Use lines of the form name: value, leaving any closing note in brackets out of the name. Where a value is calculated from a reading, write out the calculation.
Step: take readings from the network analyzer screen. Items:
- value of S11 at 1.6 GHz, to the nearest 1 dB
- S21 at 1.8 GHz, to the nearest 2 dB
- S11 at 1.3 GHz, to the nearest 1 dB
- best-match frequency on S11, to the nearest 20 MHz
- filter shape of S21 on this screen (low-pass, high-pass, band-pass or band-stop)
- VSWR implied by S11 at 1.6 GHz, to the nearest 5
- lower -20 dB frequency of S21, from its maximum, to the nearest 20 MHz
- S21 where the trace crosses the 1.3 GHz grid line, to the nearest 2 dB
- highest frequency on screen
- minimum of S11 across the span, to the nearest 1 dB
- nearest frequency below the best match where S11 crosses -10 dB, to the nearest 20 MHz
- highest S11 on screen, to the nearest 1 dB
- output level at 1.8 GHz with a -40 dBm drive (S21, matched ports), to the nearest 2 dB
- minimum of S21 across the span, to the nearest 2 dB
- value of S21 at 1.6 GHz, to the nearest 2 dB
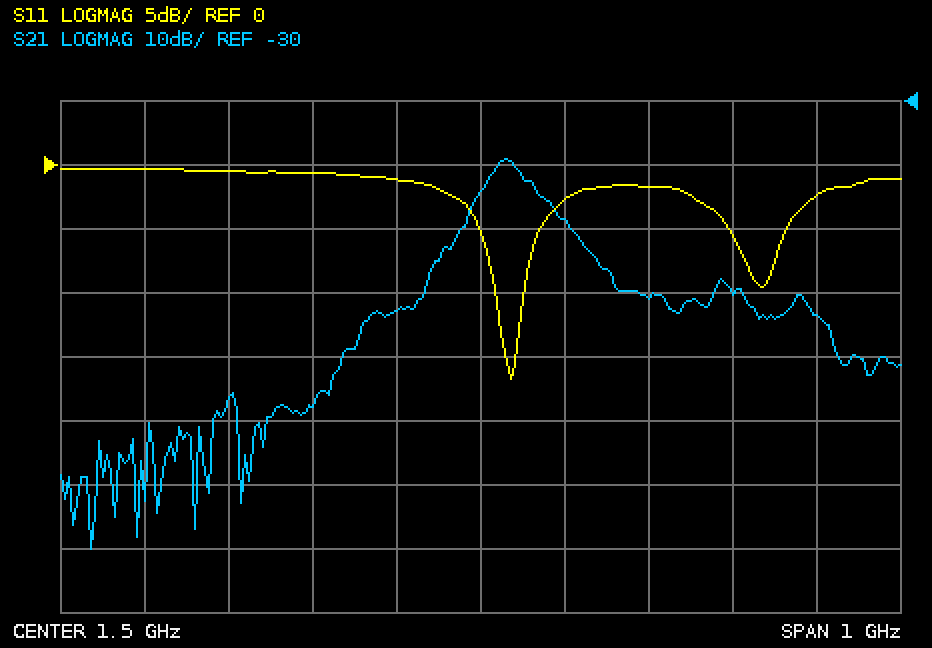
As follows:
value of S11 at 1.6 GHz, to the nearest 1 dB: -3 dB
S21 at 1.8 GHz, to the nearest 2 dB: -60 dB
S11 at 1.3 GHz, to the nearest 1 dB: -1 dB
best-match frequency on S11, to the nearest 20 MHz: 1.54 GHz
filter shape of S21 on this screen: band-pass
VSWR implied by S11 at 1.6 GHz, to the nearest 5: |Γ| = 10^(-3/20) = 0.7079; VSWR = (1 + 0.7079)/(1 − 0.7079) ≈ 5.85, so 5 to the nearest 5
lower -20 dB frequency of S21, from its maximum, to the nearest 20 MHz: 1.44 GHz
S21 where the trace crosses the 1.3 GHz grid line, to the nearest 2 dB: -78 dB
highest frequency on screen: 2 GHz
minimum of S11 across the span, to the nearest 1 dB: -17 dB
nearest frequency below the best match where S11 crosses -10 dB, to the nearest 20 MHz: 1.52 GHz
highest S11 on screen, to the nearest 1 dB: 0 dB
output level at 1.8 GHz with a -40 dBm drive (S21, matched ports), to the nearest 2 dB: -40 dBm + (-60 dB) = -100 dBm
minimum of S21 across the span, to the nearest 2 dB: -100 dB
value of S21 at 1.6 GHz, to the nearest 2 dB: -48 dB
